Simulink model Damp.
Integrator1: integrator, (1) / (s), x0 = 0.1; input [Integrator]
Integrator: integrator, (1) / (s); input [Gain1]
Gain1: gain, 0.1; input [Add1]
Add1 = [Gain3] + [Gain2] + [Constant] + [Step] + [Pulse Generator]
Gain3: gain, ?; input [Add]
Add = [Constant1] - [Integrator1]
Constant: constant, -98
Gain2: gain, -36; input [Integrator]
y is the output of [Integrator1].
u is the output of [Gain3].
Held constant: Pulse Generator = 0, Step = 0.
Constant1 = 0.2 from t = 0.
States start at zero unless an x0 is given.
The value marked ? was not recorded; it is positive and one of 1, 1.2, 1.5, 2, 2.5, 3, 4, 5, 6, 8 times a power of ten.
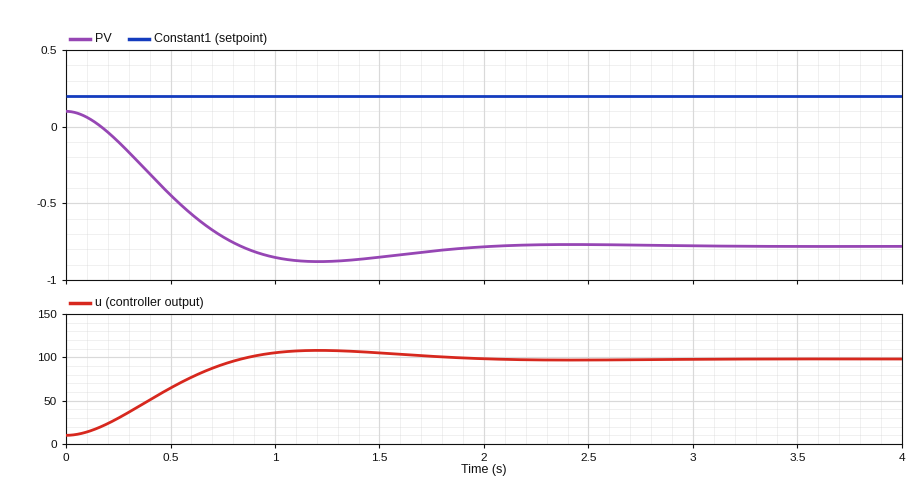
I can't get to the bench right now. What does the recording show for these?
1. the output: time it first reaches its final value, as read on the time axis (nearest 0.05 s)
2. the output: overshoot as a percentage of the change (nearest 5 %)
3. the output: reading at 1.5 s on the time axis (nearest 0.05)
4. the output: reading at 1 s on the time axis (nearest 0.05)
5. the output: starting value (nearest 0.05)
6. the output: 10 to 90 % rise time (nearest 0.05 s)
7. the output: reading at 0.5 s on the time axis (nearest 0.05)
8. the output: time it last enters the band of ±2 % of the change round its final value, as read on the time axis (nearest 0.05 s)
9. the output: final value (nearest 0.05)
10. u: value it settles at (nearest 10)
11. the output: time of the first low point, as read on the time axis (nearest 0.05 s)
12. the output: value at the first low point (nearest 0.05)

0.85 s
10 %
-0.85
-0.85
0.10
0.55 s
-0.45
1.85 s
-0.80
100
1.20 s
-0.90
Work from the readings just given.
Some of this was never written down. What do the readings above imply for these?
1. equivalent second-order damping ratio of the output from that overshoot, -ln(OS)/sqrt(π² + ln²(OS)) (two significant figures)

0.59
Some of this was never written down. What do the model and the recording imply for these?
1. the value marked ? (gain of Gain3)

100
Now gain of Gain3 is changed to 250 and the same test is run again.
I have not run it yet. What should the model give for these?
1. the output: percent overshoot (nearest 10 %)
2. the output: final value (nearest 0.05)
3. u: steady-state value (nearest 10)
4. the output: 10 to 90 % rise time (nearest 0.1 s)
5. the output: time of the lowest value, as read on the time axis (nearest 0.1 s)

30 %
-0.20
100
0.3 s
0.7 s
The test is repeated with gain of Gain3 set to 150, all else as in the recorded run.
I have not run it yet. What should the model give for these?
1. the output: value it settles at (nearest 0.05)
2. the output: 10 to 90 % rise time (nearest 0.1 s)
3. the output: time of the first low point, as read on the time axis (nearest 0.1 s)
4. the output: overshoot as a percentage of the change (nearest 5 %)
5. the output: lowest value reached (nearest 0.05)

-0.45
0.4 s
0.9 s
20 %
-0.55
